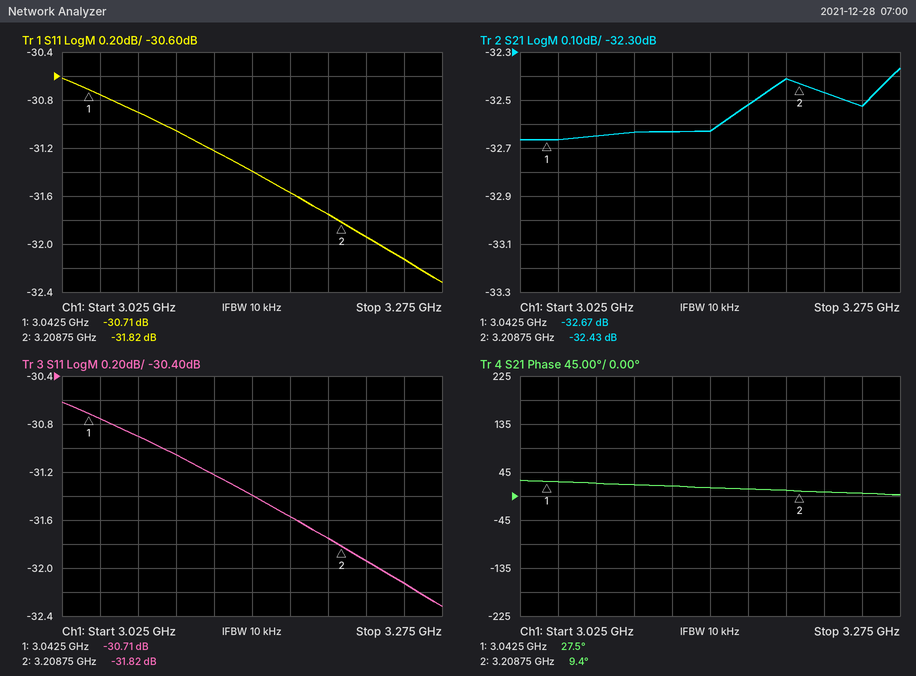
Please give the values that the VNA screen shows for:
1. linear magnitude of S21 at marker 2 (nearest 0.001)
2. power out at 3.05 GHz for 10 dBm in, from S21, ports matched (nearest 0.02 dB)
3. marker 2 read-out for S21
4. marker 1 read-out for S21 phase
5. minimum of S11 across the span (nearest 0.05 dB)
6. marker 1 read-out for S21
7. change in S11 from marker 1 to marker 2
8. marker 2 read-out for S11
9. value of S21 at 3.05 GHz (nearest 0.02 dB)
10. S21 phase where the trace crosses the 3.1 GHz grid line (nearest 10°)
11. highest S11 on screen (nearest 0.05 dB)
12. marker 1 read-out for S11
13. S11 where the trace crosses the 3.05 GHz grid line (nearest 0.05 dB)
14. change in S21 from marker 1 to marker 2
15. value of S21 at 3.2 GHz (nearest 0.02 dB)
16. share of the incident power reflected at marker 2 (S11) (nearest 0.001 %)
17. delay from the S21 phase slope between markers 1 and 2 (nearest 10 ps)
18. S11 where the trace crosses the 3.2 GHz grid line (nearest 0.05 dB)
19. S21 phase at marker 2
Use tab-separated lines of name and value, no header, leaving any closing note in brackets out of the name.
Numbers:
linear magnitude of S21 at marker 2	0.024
power out at 3.05 GHz for 10 dBm in, from S21, ports matched	-22.66 dBm
marker 2 read-out for S21	-32.43 dB
marker 1 read-out for S21 phase	27.5°
minimum of S11 across the span	-32.30 dB
marker 1 read-out for S21	-32.67 dB
change in S11 from marker 1 to marker 2	-1.11 dB
marker 2 read-out for S11	-31.82 dB
value of S21 at 3.05 GHz	-32.66 dB
S21 phase where the trace crosses the 3.1 GHz grid line	20°
highest S11 on screen	-30.60 dB
marker 1 read-out for S11	-30.71 dB
S11 where the trace crosses the 3.05 GHz grid line	-30.75 dB
change in S21 from marker 1 to marker 2	0.24 dB
value of S21 at 3.2 GHz	-32.42 dB
share of the incident power reflected at marker 2 (S11)	0.066 %
delay from the S21 phase slope between markers 1 and 2	300 ps
S11 where the trace crosses the 3.2 GHz grid line	-31.75 dB
S21 phase at marker 2	9.4°
